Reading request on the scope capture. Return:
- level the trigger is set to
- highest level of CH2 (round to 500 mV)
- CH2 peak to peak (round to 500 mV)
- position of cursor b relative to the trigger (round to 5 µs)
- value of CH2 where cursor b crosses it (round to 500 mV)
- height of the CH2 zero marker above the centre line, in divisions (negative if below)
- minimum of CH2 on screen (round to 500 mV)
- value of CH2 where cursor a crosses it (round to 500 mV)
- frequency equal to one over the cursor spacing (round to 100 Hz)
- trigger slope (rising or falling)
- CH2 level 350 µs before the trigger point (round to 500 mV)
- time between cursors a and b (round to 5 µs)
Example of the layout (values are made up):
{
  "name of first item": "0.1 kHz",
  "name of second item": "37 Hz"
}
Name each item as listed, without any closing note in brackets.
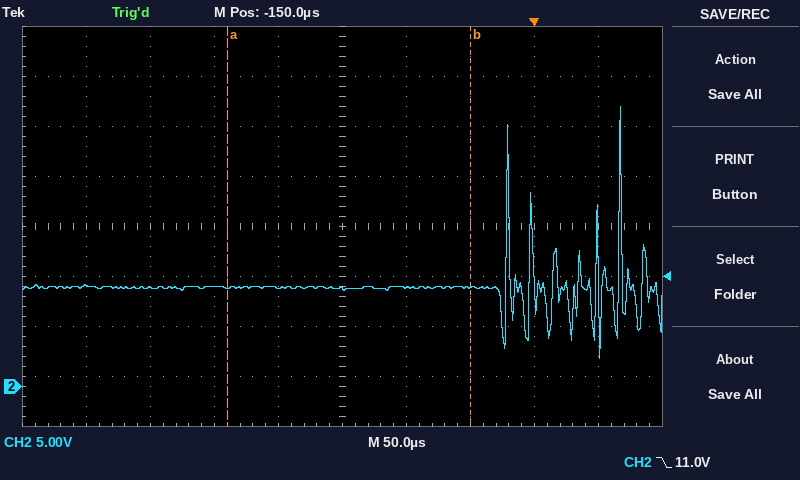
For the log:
{
  "level the trigger is set to": "11.0 V",
  "highest level of CH2": "28.0 V",
  "CH2 peak to peak": "25.0 V",
  "position of cursor b relative to the trigger": "-50 µs",
  "value of CH2 where cursor b crosses it": "10.0 V",
  "height of the CH2 zero marker above the centre line, in divisions": "-3.2 div",
  "minimum of CH2 on screen": "3.0 V",
  "value of CH2 where cursor a crosses it": "10.0 V",
  "frequency equal to one over the cursor spacing": "5.3 kHz",
  "trigger slope": "falling",
  "CH2 level 350 µs before the trigger point": "10.0 V",
  "time between cursors a and b": "190 µs"
}
